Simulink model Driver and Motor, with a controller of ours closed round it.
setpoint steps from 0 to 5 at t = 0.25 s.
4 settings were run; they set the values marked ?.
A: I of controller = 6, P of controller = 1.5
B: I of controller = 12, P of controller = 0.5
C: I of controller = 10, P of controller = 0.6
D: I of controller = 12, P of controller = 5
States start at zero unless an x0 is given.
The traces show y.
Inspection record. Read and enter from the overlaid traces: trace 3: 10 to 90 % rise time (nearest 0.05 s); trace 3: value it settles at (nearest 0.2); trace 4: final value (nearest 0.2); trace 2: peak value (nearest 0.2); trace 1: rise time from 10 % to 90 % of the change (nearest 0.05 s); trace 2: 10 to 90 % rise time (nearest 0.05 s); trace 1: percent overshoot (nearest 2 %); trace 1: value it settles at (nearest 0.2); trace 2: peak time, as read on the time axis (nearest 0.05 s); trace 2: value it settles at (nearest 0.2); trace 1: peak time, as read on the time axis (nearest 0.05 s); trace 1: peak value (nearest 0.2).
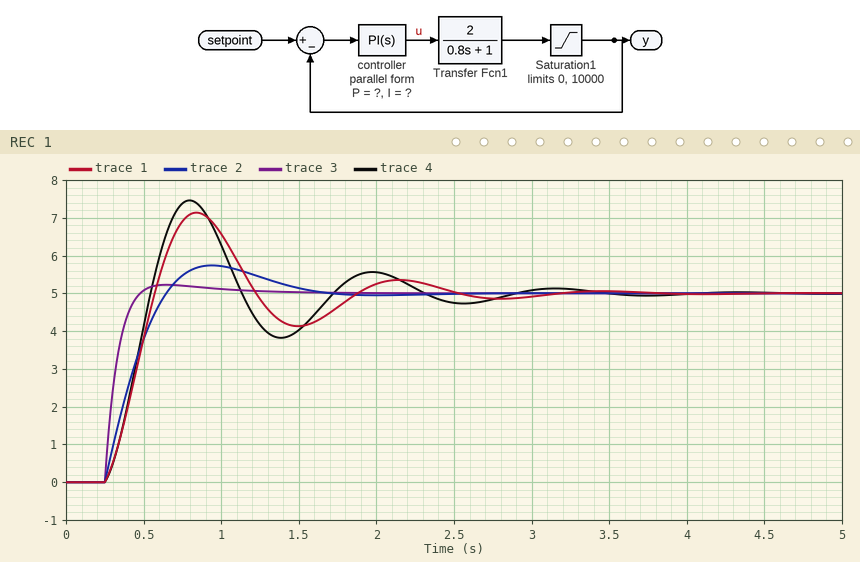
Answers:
0.15 s
5.0
5.0
5.8
0.25 s
0.30 s
42 %
5.0
0.95 s
5.0
0.85 s
7.2
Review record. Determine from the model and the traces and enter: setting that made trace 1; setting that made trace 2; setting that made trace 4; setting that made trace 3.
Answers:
C
A
B
D
